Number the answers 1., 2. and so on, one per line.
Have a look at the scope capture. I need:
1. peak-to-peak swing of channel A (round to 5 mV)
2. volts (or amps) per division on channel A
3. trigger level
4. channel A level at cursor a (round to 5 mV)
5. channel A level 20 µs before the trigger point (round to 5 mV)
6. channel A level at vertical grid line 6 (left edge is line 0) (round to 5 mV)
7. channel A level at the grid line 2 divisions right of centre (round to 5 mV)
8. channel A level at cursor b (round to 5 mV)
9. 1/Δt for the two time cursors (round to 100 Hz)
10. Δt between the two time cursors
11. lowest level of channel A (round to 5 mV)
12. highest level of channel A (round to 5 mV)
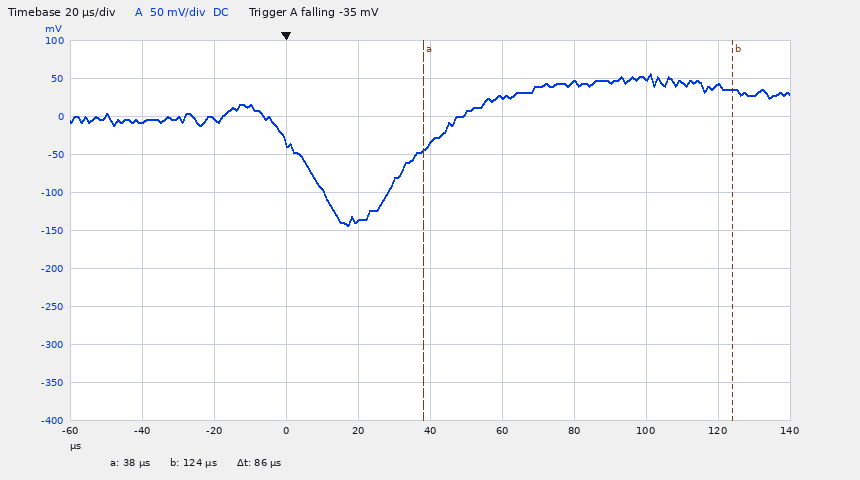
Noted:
1. 200 mV
2. 50 mV
3. -35 mV
4. -45 mV
5. -5 mV
6. 25 mV
7. 45 mV
8. 35 mV
9. 11.6 kHz
10. 86 µs
11. -145 mV
12. 55 mV
